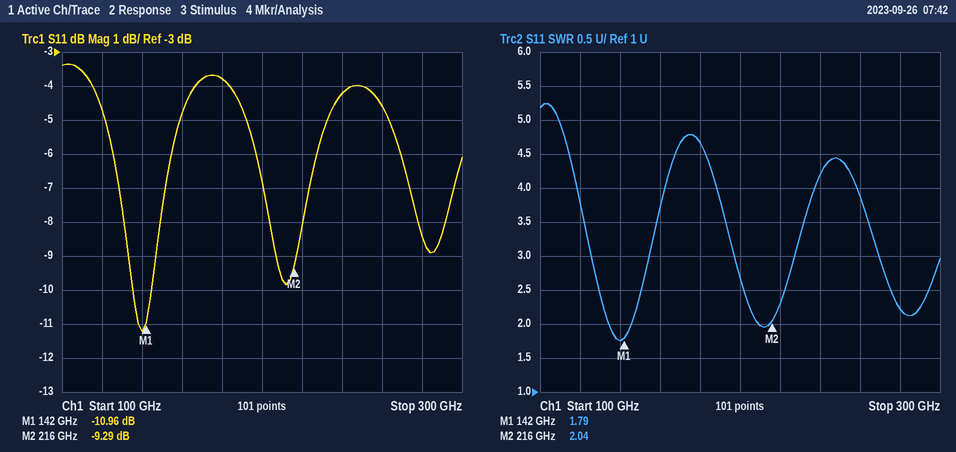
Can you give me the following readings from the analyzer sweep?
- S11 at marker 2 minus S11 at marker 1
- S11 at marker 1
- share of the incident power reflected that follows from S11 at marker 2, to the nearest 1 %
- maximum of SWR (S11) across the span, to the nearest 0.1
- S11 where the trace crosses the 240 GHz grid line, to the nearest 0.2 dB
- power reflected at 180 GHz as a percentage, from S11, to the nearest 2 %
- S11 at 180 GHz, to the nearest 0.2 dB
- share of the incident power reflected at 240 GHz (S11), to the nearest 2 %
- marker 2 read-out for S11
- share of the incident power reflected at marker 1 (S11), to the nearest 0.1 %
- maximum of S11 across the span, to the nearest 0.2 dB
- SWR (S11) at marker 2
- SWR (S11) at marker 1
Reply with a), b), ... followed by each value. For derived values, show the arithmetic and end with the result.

a) -9.29 − (-10.96) = 1.67 dB
b) -10.96 dB
c) 10^(-9.29/10) ≈ 12 %
d) 5.2
e) -4.2 dB
f) 10^(-3.8/10) ≈ 42 %
g) -3.8 dB
h) 10^(-4.2/10) ≈ 38 %
i) -9.29 dB
j) 10^(-10.96/10) ≈ 8.0 %
k) -3.4 dB
l) 2.04
m) 1.79
